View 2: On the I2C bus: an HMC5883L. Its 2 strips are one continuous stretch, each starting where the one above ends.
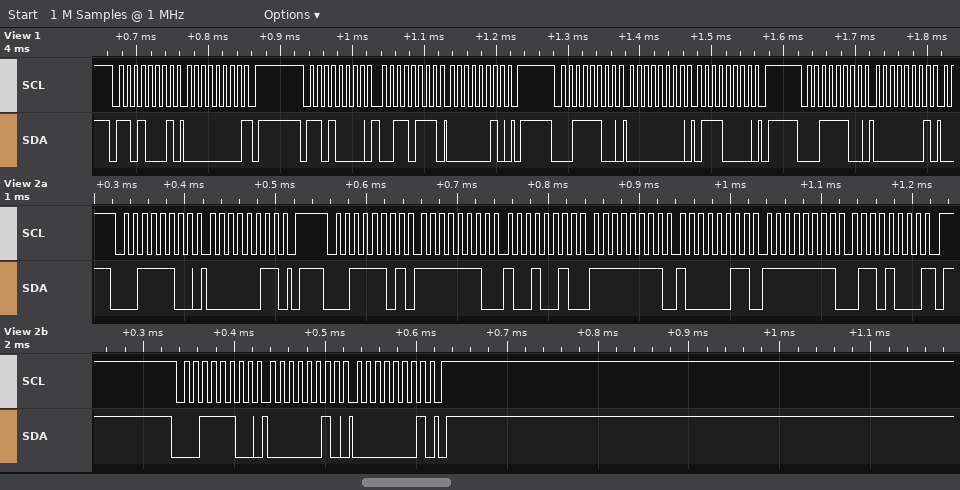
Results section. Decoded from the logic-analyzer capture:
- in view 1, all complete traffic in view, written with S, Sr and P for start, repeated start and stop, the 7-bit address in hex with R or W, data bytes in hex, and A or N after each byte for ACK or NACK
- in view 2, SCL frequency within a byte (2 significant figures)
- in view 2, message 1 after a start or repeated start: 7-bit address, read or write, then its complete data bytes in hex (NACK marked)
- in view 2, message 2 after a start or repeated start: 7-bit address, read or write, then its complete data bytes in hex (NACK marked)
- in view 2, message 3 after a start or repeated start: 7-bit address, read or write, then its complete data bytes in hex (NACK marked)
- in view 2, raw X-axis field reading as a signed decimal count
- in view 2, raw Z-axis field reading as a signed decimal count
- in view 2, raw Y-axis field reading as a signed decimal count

S 68R A 00 N P S 68W A 37 A 02 A P S 1EW A 00 A 70 A P S 1EW A 01 A
100 kHz
0x1E write: 03
0x1E read: FE 92 FF 83 FF 68 NACK
0x1E write: 02 01
-366
-125
-152
